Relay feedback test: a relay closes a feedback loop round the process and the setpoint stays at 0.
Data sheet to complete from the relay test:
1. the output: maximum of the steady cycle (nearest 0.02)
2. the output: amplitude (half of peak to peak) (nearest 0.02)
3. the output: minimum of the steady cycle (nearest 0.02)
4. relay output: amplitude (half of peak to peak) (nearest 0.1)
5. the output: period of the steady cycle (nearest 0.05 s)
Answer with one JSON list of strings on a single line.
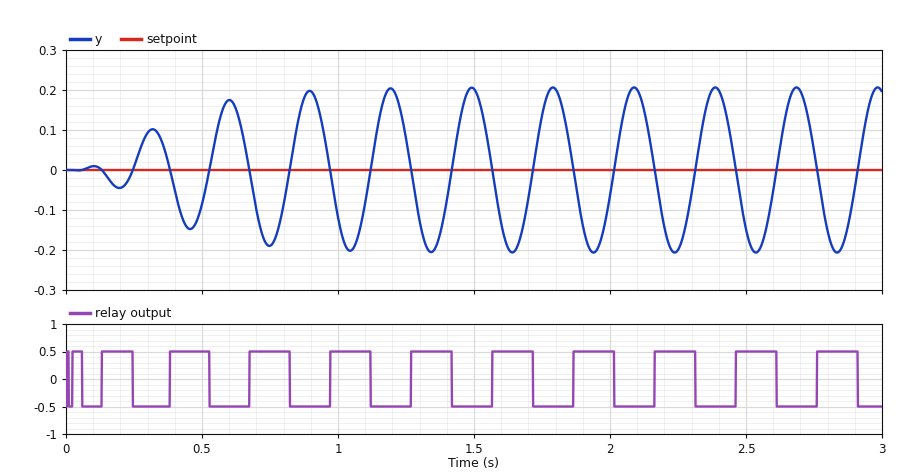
["0.20", "0.20", "-0.20", "0.5", "0.30 s"]
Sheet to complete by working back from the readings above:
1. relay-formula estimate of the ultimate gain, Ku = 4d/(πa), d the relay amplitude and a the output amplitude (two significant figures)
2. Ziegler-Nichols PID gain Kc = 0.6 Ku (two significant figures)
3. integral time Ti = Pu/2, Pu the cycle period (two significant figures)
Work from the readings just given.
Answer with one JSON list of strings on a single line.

["3.2", "1.9", "0.15 s"]
